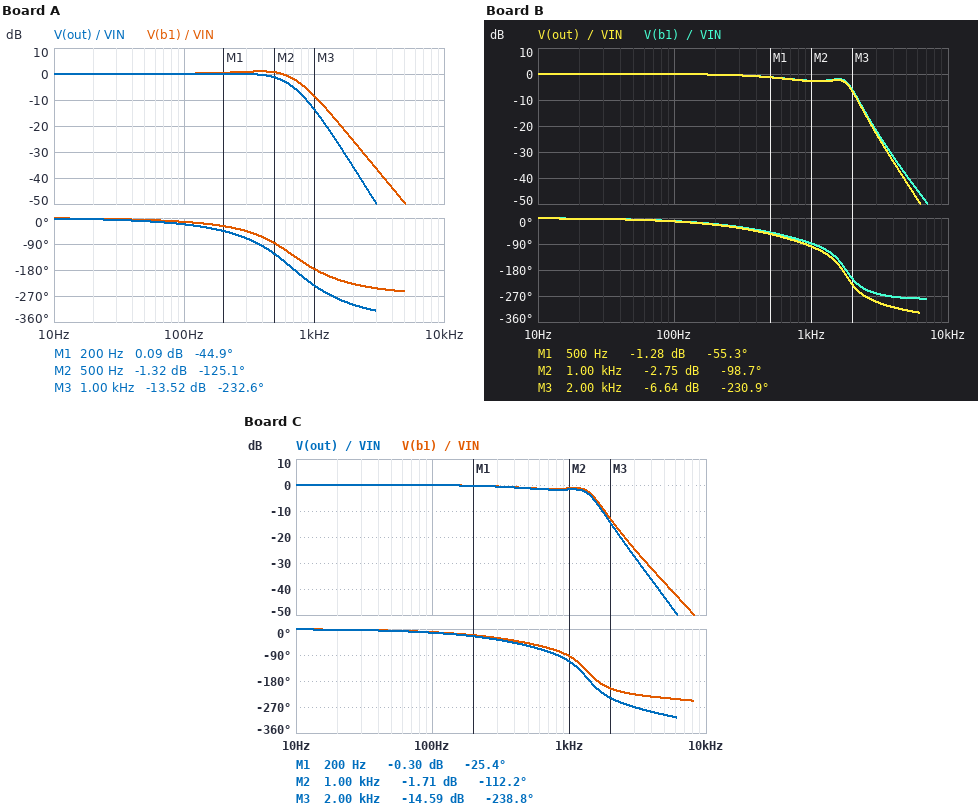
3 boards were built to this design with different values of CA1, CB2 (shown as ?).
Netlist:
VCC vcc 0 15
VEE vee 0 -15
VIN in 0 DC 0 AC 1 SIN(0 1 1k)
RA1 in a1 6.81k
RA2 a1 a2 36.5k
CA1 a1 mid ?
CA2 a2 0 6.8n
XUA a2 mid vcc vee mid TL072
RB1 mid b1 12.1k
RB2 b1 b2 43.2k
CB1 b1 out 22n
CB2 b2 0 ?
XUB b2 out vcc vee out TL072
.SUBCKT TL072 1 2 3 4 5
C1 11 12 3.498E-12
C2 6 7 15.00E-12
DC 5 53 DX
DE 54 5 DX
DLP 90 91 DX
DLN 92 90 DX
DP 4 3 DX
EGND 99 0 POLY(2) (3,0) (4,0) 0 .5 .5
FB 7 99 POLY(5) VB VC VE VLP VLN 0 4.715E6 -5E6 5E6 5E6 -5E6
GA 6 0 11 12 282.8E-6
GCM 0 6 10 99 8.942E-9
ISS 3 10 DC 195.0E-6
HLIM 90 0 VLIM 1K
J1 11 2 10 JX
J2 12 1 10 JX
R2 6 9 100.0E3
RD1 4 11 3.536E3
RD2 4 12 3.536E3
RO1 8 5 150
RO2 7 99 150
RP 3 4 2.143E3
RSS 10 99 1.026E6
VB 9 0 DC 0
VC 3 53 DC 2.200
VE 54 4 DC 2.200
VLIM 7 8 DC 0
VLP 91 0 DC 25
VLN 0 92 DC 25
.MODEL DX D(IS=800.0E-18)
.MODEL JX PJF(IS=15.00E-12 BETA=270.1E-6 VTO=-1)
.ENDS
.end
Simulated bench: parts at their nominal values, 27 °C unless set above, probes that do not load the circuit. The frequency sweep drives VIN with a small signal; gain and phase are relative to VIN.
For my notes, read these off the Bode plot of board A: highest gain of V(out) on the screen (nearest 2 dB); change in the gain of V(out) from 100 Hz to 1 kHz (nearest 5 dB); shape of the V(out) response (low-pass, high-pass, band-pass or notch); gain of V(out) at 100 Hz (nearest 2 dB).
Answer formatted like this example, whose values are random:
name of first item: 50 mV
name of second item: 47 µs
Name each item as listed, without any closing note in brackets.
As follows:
highest gain of V(out) on the screen: 0 dB
change in the gain of V(out) from 100 Hz to 1 kHz: -15 dB
shape of the V(out) response: low-pass
gain of V(out) at 100 Hz: 0 dB
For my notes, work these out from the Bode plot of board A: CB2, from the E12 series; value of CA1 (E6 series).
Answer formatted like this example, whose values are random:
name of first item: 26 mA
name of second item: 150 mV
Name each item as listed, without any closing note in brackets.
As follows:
CB2, from the E12 series: 5.6 nF
value of CA1: 22 nF
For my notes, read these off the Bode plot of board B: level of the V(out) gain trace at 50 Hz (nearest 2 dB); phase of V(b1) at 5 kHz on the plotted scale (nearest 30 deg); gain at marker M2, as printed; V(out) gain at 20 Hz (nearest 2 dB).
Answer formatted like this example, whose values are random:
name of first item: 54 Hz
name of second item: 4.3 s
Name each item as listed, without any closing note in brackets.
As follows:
level of the V(out) gain trace at 50 Hz: 0 dB
phase of V(b1) at 5 kHz on the plotted scale: -270 deg
gain at marker M2, as printed: -2.75 dB
V(out) gain at 20 Hz: 0 dB
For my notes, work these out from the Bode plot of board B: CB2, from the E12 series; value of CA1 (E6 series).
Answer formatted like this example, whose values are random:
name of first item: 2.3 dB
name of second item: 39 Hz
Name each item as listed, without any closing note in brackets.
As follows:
CB2, from the E12 series: 680 pF
value of CA1: 10 nF
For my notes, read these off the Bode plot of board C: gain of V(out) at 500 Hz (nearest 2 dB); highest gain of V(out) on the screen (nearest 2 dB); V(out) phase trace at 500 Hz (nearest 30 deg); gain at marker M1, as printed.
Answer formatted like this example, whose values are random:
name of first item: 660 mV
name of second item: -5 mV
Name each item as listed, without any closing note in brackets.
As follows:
gain of V(out) at 500 Hz: -2 dB
highest gain of V(out) on the screen: 0 dB
V(out) phase trace at 500 Hz: -60 deg
gain at marker M1, as printed: -0.30 dB
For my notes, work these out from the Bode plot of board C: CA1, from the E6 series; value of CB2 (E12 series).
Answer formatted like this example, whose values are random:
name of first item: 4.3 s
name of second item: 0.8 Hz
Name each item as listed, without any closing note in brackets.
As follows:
CA1, from the E6 series: 4.7 nF
value of CB2: 1.2 nF
